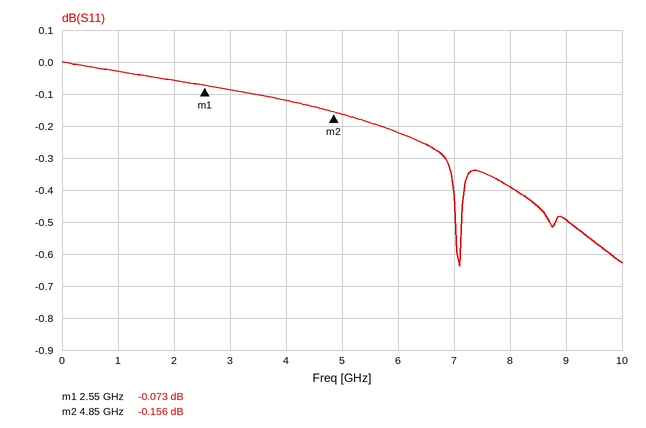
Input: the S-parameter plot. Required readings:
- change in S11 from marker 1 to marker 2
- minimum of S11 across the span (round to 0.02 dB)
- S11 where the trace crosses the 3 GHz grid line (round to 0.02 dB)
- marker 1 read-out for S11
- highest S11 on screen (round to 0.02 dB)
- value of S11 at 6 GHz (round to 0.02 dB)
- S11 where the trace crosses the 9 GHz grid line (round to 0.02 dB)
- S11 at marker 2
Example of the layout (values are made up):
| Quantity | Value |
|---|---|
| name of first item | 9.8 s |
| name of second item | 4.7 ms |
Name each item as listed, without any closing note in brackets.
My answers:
| Quantity | Value |
|---|---|
| change in S11 from marker 1 to marker 2 | -0.083 dB |
| minimum of S11 across the span | -0.64 dB |
| S11 where the trace crosses the 3 GHz grid line | -0.08 dB |
| marker 1 read-out for S11 | -0.073 dB |
| highest S11 on screen | 0.00 dB |
| value of S11 at 6 GHz | -0.22 dB |
| S11 where the trace crosses the 9 GHz grid line | -0.50 dB |
| S11 at marker 2 | -0.156 dB |
